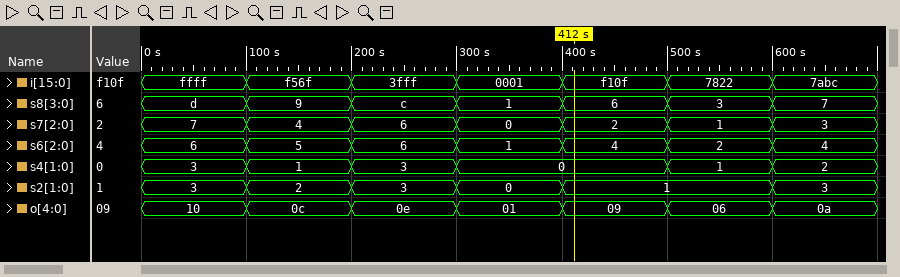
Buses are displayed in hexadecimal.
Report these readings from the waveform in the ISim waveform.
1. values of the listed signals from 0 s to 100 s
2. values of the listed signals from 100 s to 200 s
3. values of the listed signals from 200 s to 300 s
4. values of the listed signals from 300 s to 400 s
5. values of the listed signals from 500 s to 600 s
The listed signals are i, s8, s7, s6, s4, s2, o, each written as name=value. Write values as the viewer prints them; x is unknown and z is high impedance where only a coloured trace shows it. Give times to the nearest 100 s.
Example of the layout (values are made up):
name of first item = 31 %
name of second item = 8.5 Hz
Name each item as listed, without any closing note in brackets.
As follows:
values of the listed signals from 0 s to 100 s = i=ffff, s8=d, s7=7, s6=6, s4=3, s2=3, o=10
values of the listed signals from 100 s to 200 s = i=f56f, s8=9, s7=4, s6=5, s4=1, s2=2, o=0c
values of the listed signals from 200 s to 300 s = i=3fff, s8=c, s7=6, s6=6, s4=3, s2=3, o=0e
values of the listed signals from 300 s to 400 s = i=0001, s8=1, s7=0, s6=1, s4=0, s2=0, o=01
values of the listed signals from 500 s to 600 s = i=7822, s8=3, s7=1, s6=2, s4=1, s2=1, o=06
